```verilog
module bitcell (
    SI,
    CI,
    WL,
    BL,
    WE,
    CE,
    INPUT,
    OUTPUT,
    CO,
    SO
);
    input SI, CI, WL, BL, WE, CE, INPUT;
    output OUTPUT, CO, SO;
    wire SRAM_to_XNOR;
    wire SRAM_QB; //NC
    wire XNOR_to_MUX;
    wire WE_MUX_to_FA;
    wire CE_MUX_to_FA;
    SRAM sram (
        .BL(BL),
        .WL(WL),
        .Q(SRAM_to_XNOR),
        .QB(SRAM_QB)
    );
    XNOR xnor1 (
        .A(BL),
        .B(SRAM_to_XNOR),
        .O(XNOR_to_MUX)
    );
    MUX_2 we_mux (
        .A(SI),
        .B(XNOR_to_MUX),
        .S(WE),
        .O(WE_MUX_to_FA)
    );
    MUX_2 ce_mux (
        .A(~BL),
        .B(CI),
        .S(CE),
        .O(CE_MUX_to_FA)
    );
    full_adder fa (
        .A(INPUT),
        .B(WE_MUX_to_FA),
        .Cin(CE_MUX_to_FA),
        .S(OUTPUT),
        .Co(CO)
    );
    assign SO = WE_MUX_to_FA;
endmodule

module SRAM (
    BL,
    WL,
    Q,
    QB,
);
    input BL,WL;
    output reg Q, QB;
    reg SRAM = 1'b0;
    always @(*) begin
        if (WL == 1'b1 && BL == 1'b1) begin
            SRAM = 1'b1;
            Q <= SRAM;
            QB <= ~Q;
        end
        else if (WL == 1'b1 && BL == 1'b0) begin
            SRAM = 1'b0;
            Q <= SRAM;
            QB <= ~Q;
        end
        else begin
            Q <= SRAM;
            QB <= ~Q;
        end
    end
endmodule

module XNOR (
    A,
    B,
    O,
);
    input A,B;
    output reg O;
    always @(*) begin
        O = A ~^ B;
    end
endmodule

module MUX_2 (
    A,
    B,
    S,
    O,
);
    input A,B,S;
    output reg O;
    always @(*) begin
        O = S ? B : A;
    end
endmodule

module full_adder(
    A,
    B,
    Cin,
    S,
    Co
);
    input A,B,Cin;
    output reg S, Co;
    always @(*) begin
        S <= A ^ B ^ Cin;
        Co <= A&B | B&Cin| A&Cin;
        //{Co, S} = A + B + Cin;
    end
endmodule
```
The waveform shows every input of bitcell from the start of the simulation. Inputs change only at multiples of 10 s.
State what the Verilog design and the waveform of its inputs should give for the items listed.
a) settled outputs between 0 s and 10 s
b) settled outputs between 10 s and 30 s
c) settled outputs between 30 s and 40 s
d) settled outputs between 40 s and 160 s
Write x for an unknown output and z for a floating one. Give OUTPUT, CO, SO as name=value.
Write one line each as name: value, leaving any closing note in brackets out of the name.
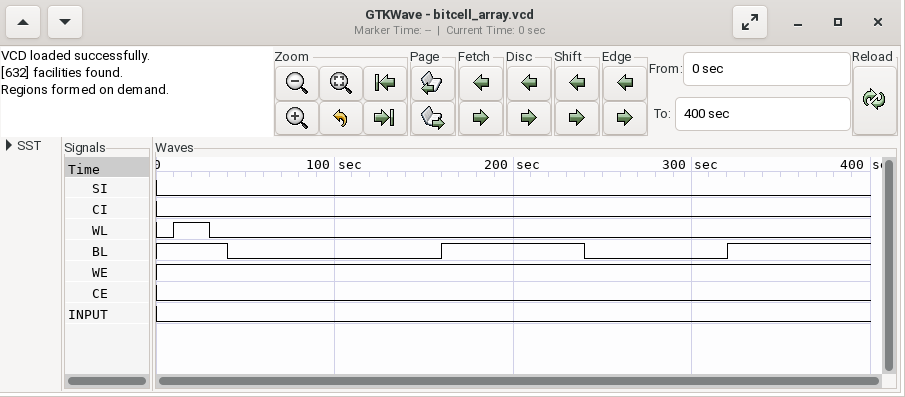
settled outputs between 0 s and 10 s: OUTPUT=0, CO=0, SO=0
settled outputs between 10 s and 30 s: OUTPUT=1, CO=0, SO=1
settled outputs between 30 s and 40 s: OUTPUT=1, CO=0, SO=1
settled outputs between 40 s and 160 s: OUTPUT=1, CO=0, SO=0
